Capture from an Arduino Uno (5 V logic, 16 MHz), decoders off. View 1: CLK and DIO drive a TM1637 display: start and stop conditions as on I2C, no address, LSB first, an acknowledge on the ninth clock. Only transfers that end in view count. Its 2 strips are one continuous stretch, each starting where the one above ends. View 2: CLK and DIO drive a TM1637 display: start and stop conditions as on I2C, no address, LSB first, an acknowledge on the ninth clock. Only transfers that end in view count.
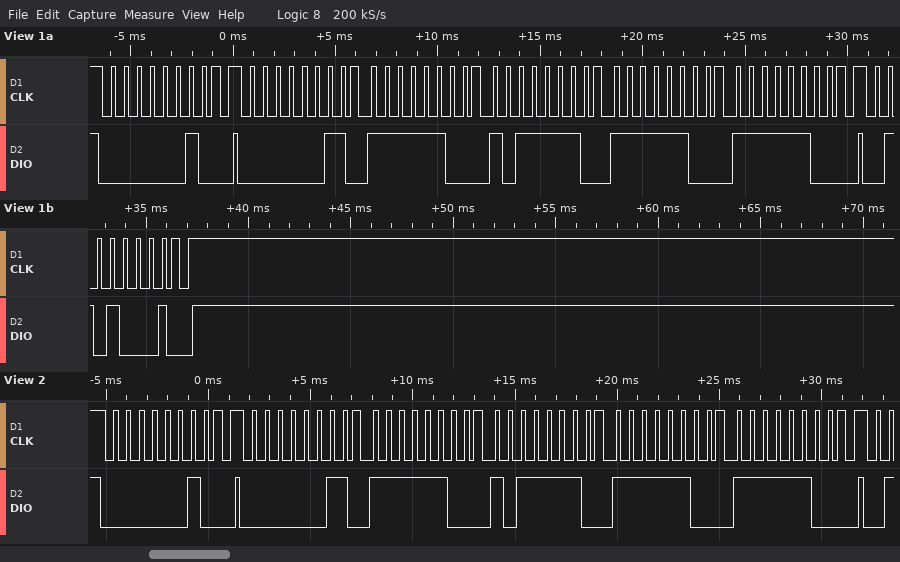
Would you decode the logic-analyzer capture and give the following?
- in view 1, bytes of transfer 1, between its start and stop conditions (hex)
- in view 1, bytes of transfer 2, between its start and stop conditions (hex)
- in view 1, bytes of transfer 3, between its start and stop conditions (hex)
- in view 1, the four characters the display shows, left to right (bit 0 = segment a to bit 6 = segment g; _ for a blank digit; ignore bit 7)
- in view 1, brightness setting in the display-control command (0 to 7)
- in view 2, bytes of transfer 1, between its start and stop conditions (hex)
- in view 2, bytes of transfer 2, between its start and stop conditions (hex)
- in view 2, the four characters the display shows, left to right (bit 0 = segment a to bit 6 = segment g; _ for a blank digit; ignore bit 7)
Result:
40
C0 3F 7D 3F 3F
8A
0600
2
40
C0 3F 7D 3F 3F
0600
